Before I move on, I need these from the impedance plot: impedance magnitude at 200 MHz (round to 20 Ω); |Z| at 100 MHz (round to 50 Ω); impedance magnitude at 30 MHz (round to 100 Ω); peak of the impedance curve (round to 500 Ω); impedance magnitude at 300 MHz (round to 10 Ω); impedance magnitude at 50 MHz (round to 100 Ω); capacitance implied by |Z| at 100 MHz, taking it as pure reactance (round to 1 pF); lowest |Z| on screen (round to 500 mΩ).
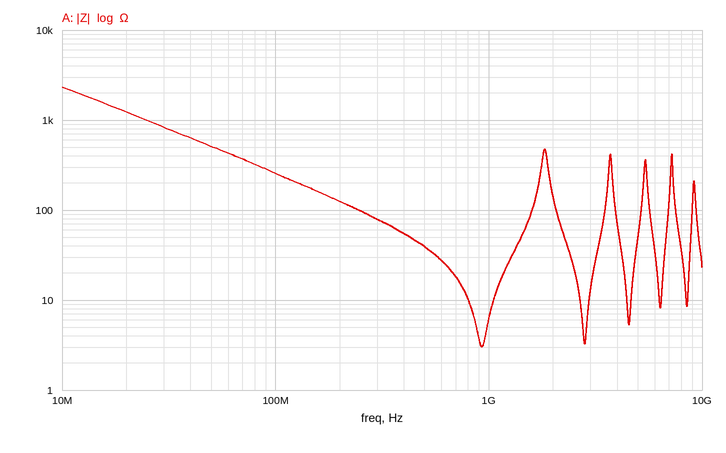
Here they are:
120 Ω
250 Ω
800 Ω
2.5 kΩ
80 Ω
500 Ω
6 pF
3.0 Ω
